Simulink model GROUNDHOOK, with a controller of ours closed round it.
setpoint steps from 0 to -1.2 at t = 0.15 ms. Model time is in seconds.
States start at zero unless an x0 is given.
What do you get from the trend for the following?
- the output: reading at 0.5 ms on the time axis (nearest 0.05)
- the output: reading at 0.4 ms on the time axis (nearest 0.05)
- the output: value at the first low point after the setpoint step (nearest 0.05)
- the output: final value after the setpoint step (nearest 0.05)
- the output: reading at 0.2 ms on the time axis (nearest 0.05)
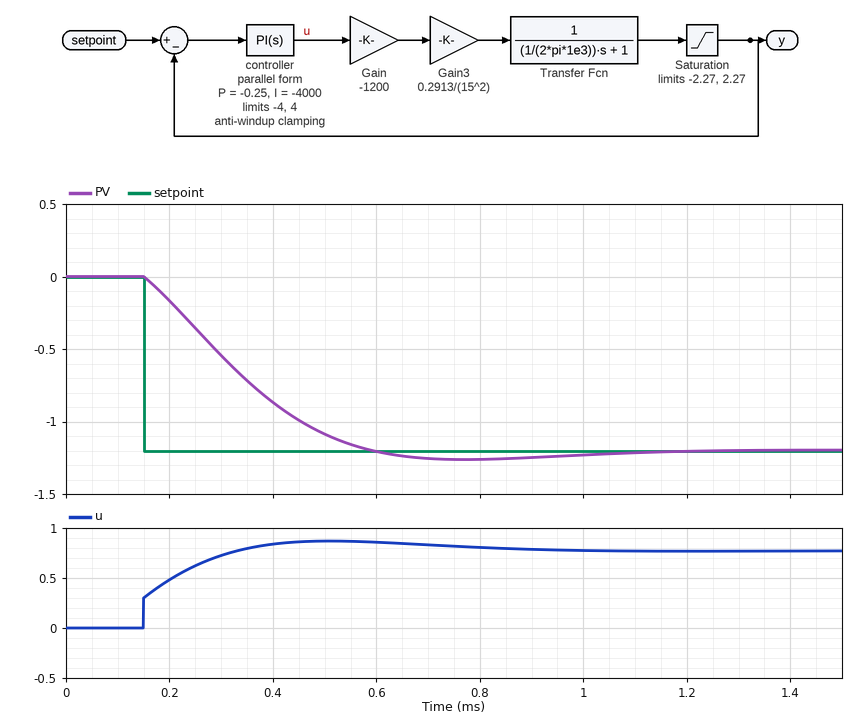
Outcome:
-1.10
-0.85
-1.25
-1.20
-0.15
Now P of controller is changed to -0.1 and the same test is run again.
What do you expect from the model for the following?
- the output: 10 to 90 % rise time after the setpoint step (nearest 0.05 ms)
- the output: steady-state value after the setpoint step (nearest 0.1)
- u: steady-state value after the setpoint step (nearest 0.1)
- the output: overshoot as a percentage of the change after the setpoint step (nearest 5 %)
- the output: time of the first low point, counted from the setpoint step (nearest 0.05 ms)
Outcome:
0.30 ms
-1.2
0.8
10 %
0.60 ms
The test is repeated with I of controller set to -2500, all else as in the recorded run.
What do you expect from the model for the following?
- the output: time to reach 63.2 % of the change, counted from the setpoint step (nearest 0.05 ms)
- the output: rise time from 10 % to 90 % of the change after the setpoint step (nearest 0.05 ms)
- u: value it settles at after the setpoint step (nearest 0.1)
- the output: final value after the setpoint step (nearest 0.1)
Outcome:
0.30 ms
0.50 ms
0.8
-1.2
